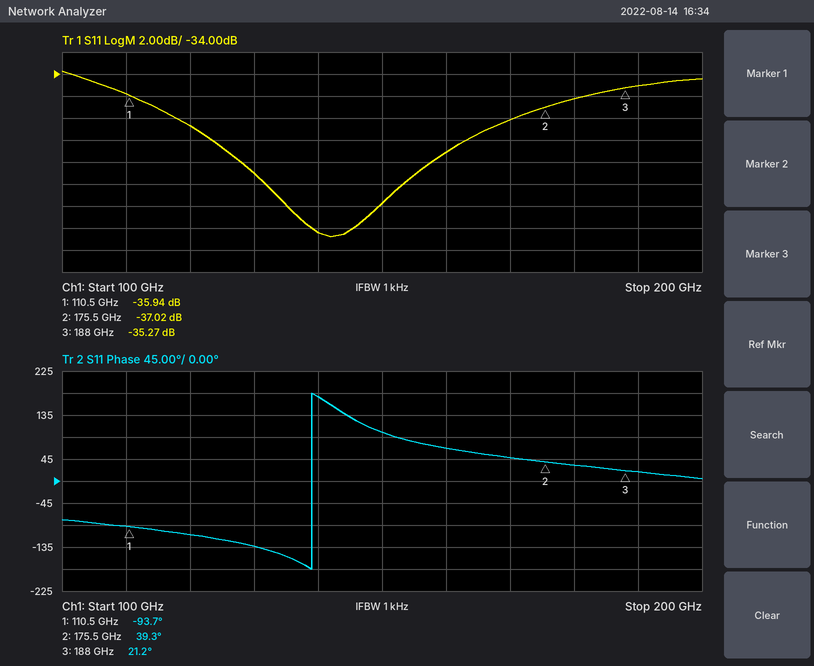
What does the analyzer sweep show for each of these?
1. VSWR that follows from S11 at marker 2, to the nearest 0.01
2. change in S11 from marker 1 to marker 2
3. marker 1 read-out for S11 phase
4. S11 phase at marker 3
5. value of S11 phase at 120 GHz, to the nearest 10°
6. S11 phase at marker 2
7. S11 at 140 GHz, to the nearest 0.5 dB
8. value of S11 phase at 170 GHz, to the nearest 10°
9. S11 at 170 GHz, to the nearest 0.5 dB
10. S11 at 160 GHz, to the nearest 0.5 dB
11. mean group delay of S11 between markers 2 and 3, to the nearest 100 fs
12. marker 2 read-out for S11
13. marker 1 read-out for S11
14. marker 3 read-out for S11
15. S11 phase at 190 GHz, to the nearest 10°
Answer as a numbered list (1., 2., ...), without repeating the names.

1. 1.03
2. -1.08 dB
3. -93.7°
4. 21.2°
5. -110°
6. 39.3°
7. -48.5 dB
8. 50°
9. -38.0 dB
10. -41.0 dB
11. 4.0 ps
12. -37.02 dB
13. -35.94 dB
14. -35.27 dB
15. 20°
